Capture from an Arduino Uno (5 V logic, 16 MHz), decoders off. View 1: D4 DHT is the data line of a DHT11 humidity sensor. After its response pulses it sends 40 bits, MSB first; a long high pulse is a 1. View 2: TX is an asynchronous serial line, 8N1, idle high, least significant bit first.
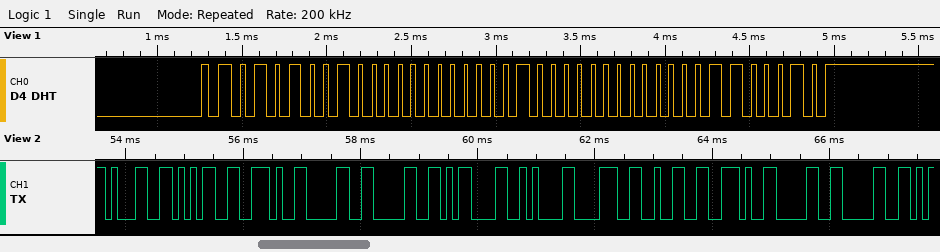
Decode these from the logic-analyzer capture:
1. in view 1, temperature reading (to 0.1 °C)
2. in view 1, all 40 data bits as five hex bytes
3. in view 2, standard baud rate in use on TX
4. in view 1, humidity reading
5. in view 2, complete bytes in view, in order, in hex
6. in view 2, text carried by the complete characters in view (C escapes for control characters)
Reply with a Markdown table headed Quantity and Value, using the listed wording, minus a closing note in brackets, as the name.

| Quantity | Value |
|---|---|
| in view 1, temperature reading | 16.0 °C |
| in view 1, all 40 data bits as five hex bytes | 52 00 10 00 62 |
| in view 2, standard baud rate in use on TX | 9600 baud |
| in view 1, humidity reading | 82 % |
| in view 2, complete bytes in view, in order, in hex | 31 35 2E 30 30 0D 0A 38 32 2E 30 30 |
| in view 2, text carried by the complete characters in view | "15.00\r\n82.00" |
